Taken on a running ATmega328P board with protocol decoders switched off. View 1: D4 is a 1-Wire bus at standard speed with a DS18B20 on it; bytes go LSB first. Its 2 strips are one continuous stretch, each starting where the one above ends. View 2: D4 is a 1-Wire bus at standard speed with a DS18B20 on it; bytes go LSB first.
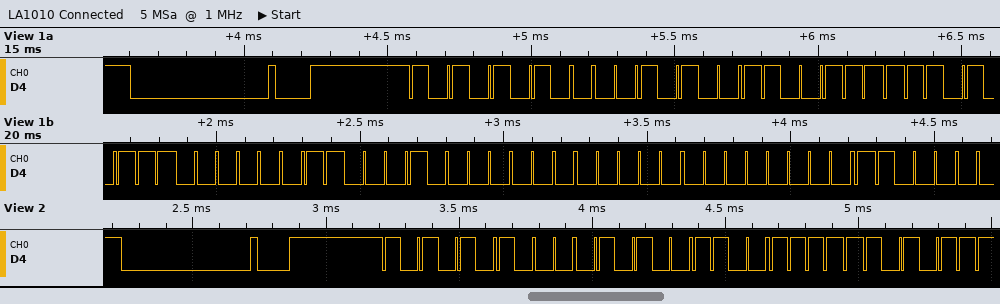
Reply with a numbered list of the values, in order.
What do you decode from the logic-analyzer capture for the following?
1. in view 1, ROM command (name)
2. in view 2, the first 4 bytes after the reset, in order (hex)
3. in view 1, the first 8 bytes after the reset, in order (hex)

1. Match ROM
2. 55 28 F3 EB
3. 55 28 F3 EB C0 08 00 00
